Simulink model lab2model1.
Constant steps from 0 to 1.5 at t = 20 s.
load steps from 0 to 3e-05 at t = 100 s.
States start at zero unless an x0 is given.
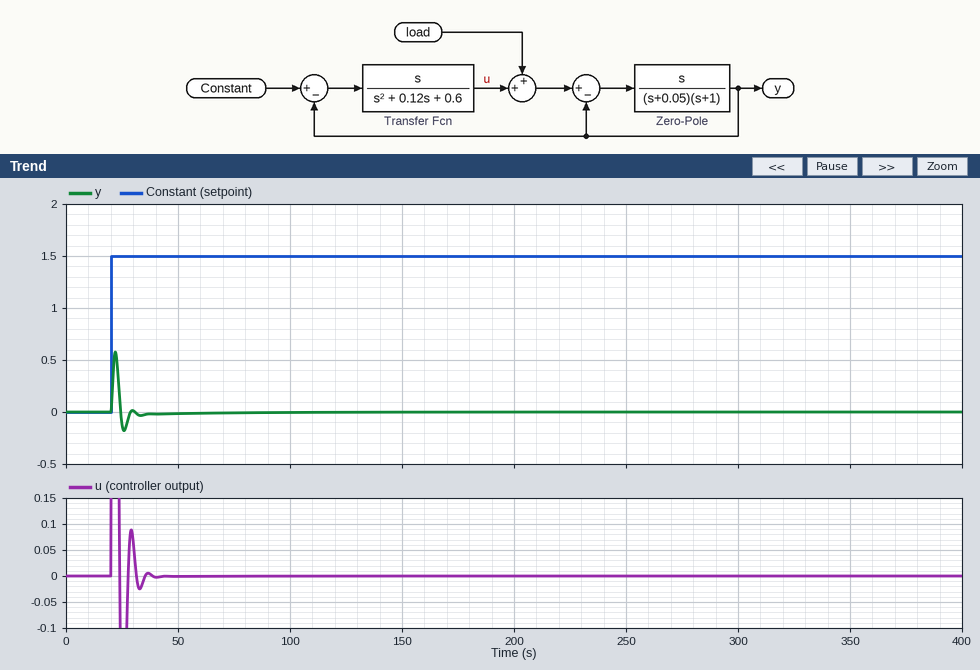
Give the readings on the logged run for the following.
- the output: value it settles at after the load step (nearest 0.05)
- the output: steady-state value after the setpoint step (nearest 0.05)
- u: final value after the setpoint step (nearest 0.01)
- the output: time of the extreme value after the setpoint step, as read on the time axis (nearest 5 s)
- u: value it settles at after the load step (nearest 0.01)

0.00
0.00
0.00
20 s
0.00
